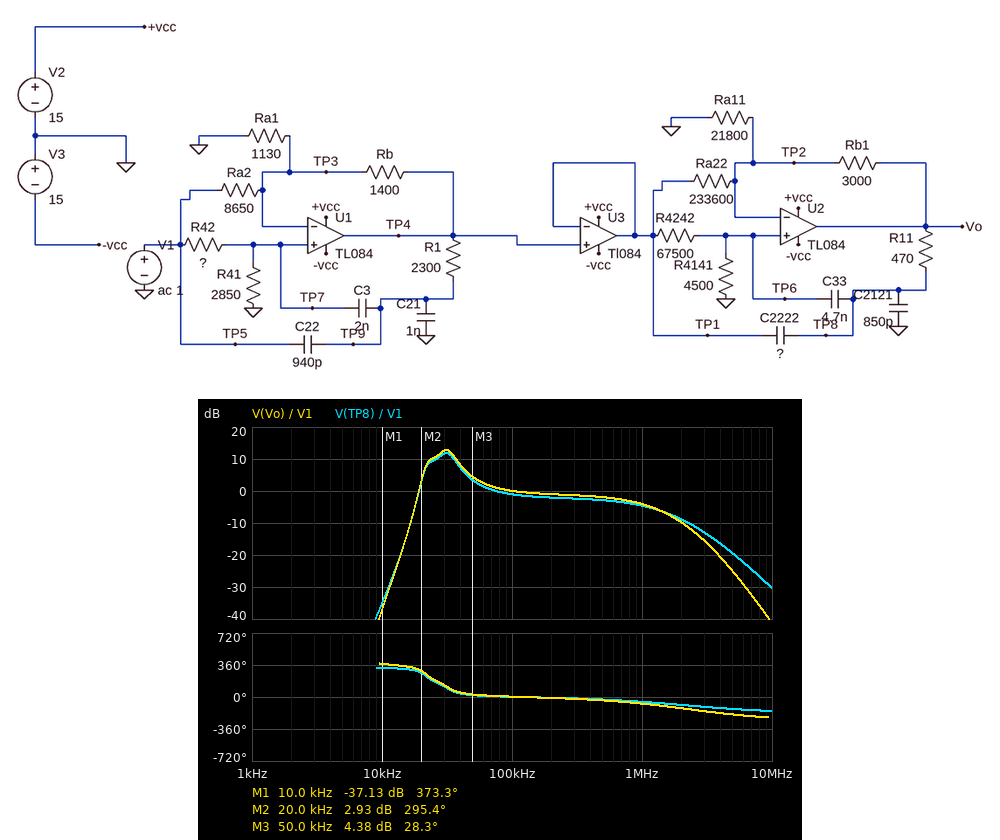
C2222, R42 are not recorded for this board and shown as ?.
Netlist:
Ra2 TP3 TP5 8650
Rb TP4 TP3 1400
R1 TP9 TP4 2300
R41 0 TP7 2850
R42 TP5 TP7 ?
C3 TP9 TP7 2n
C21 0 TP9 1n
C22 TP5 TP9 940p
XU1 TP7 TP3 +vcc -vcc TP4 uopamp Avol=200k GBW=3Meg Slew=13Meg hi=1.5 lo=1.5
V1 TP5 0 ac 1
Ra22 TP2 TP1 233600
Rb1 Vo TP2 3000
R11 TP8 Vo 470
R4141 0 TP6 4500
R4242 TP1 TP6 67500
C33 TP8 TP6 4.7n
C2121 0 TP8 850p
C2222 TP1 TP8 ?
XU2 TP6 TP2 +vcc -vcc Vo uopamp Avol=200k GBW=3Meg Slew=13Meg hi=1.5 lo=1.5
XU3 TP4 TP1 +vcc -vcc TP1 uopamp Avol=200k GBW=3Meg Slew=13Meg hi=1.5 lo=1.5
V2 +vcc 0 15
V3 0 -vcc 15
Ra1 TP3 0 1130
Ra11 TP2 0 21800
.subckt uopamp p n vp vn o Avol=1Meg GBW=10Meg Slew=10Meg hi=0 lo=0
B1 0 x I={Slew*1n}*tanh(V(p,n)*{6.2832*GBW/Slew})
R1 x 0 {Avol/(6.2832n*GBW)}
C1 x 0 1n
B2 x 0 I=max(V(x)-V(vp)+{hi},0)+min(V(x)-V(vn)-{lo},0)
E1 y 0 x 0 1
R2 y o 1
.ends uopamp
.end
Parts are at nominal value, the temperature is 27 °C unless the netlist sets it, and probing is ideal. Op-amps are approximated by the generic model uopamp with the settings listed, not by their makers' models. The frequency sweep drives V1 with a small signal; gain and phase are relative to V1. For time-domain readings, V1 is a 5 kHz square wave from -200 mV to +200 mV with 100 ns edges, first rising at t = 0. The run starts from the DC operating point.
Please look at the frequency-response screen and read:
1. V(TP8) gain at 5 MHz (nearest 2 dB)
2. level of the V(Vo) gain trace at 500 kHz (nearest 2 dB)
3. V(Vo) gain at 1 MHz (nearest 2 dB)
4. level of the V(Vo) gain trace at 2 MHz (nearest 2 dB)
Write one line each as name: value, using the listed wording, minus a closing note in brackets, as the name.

V(TP8) gain at 5 MHz: -20 dB
level of the V(Vo) gain trace at 500 kHz: -2 dB
V(Vo) gain at 1 MHz: -4 dB
level of the V(Vo) gain trace at 2 MHz: -10 dB
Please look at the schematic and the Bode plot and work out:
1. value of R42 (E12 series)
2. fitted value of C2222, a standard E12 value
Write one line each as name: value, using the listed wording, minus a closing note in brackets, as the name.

value of R42: 33 kΩ
fitted value of C2222, a standard E12 value: 4.7 nF
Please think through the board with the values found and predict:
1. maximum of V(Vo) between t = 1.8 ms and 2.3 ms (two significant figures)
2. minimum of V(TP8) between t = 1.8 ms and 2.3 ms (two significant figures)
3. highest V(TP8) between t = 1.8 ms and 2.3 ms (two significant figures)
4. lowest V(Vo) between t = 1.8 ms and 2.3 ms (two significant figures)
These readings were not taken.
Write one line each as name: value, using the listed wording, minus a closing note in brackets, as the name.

maximum of V(Vo) between t = 1.8 ms and 2.3 ms: 330 mV
minimum of V(TP8) between t = 1.8 ms and 2.3 ms: -310 mV
highest V(TP8) between t = 1.8 ms and 2.3 ms: 310 mV
lowest V(Vo) between t = 1.8 ms and 2.3 ms: -330 mV
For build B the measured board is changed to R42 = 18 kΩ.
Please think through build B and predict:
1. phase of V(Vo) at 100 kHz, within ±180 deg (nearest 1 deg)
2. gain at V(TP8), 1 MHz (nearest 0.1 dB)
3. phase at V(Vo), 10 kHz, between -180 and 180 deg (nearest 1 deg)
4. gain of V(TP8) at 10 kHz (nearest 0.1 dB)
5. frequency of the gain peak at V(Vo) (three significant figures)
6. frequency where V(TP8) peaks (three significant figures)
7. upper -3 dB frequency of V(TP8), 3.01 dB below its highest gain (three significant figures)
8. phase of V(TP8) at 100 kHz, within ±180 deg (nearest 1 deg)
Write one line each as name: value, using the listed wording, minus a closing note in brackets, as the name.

phase of V(Vo) at 100 kHz, within ±180 deg: 1 deg
gain at V(TP8), 1 MHz: -4.6 dB
phase at V(Vo), 10 kHz, between -180 and 180 deg: -169 deg
gain of V(TP8) at 10 kHz: -33.3 dB
frequency of the gain peak at V(Vo): 33.0 kHz
frequency where V(TP8) peaks: 32.9 kHz
upper -3 dB frequency of V(TP8), 3.01 dB below its highest gain: 42.6 kHz
phase of V(TP8) at 100 kHz, within ±180 deg: -1 deg
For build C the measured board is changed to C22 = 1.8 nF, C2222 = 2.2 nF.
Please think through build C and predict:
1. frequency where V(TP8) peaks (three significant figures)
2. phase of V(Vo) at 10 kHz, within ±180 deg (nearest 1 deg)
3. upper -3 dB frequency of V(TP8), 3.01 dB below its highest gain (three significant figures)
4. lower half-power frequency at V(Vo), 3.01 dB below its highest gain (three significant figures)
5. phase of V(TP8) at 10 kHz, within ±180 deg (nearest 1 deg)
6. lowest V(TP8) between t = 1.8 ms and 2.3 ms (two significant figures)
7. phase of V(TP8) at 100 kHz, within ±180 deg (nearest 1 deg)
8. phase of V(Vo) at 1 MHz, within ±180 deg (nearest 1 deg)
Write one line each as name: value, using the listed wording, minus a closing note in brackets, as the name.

frequency where V(TP8) peaks: 29.3 kHz
phase of V(Vo) at 10 kHz, within ±180 deg: -2 deg
upper -3 dB frequency of V(TP8), 3.01 dB below its highest gain: 31.2 kHz
lower half-power frequency at V(Vo), 3.01 dB below its highest gain: 27.7 kHz
phase of V(TP8) at 10 kHz, within ±180 deg: -75 deg
lowest V(TP8) between t = 1.8 ms and 2.3 ms: -280 mV
phase of V(TP8) at 100 kHz, within ±180 deg: 3 deg
phase of V(Vo) at 1 MHz, within ±180 deg: -75 deg
